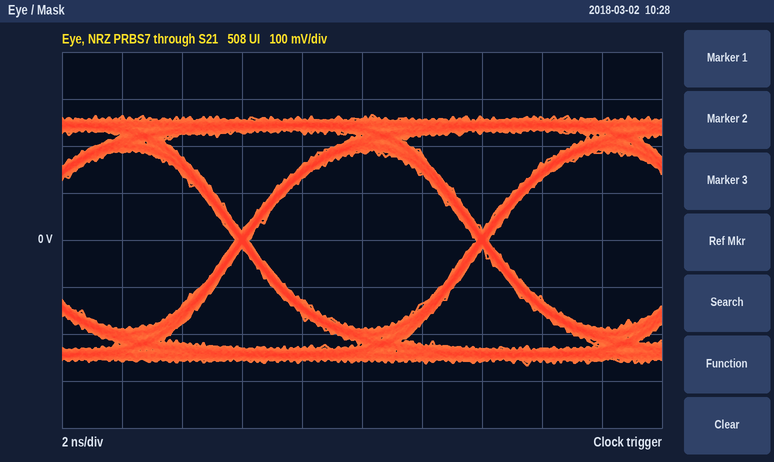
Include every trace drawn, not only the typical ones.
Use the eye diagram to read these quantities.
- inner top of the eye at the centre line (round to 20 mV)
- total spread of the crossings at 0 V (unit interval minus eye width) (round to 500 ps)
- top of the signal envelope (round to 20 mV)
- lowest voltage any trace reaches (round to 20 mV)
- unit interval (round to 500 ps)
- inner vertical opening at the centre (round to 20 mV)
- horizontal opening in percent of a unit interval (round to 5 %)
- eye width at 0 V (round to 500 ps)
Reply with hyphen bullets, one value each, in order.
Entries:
- 180 mV
- 500 ps
- 260 mV
- -260 mV
- 8.0 ns
- 380 mV
- 95 %
- 7.5 ns
